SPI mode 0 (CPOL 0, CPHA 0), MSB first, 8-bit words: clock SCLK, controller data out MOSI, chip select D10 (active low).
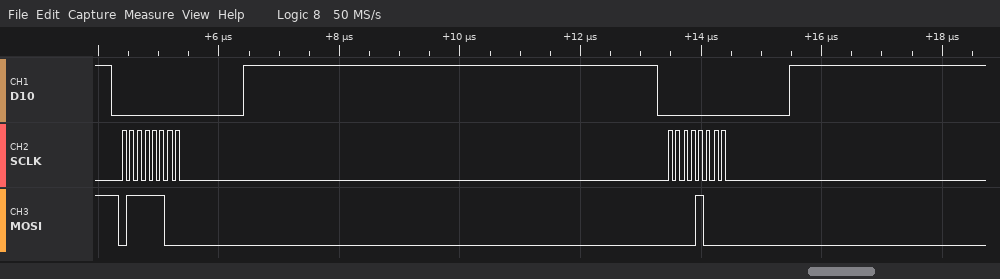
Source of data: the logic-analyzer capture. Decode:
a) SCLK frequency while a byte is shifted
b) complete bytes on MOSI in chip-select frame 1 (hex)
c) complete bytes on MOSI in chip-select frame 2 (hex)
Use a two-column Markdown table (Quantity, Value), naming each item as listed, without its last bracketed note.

| Quantity | Value |
|---|---|
| SCLK frequency while a byte is shifted | 8 MHz |
| complete bytes on MOSI in chip-select frame 1 | 7C |
| complete bytes on MOSI in chip-select frame 2 | 08 |
